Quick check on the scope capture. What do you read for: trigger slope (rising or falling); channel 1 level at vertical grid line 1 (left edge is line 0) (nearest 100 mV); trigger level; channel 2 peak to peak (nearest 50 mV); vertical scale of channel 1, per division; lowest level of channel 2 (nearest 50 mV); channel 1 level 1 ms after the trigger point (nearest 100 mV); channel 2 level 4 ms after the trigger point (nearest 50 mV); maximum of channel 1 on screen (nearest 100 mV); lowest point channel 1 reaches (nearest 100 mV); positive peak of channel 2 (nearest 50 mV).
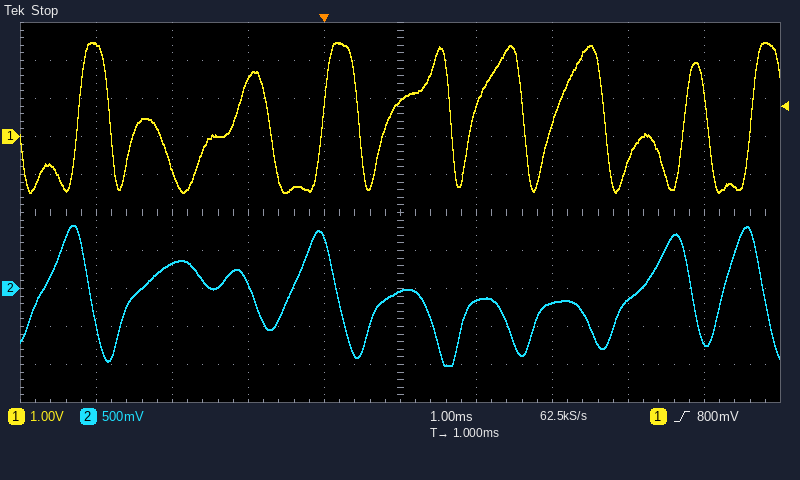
rising
2.4 V
800 mV
1.85 V
1 V
-1.00 V
900 mV
-150 mV
2.5 V
-1.5 V
850 mV
